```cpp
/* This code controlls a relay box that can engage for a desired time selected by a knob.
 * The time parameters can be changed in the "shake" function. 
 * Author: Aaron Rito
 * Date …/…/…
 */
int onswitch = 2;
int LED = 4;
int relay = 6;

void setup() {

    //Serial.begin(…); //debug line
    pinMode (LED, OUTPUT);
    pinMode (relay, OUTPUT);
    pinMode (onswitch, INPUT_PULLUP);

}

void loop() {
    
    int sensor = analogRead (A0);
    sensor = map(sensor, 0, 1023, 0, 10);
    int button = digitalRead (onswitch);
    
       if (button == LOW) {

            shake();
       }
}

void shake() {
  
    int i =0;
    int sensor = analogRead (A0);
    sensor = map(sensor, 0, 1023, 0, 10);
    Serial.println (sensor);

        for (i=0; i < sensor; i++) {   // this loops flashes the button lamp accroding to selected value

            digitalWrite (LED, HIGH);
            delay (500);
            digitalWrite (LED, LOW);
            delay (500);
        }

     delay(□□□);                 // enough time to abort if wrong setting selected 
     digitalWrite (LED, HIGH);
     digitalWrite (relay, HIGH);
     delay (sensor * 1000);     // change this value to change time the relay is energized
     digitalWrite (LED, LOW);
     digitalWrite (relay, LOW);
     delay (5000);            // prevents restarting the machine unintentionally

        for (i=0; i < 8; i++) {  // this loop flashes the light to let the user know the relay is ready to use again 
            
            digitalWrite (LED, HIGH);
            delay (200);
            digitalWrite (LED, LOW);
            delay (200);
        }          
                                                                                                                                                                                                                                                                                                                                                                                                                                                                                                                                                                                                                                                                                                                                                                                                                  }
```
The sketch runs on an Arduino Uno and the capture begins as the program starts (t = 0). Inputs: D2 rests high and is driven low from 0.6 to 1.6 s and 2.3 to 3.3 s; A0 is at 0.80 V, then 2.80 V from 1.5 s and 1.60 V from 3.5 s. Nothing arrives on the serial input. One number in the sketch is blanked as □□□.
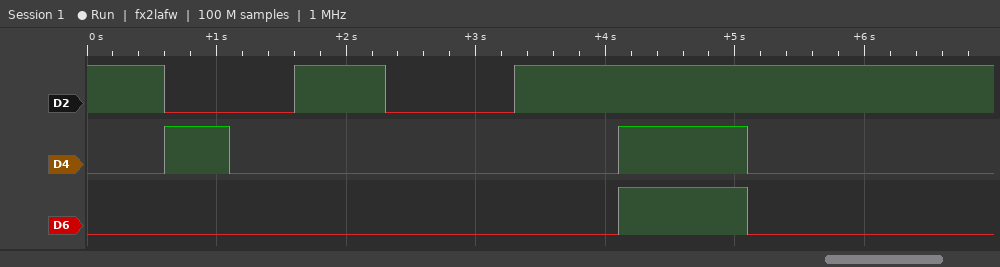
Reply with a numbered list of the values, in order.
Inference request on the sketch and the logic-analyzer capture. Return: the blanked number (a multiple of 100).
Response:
1. 2500
